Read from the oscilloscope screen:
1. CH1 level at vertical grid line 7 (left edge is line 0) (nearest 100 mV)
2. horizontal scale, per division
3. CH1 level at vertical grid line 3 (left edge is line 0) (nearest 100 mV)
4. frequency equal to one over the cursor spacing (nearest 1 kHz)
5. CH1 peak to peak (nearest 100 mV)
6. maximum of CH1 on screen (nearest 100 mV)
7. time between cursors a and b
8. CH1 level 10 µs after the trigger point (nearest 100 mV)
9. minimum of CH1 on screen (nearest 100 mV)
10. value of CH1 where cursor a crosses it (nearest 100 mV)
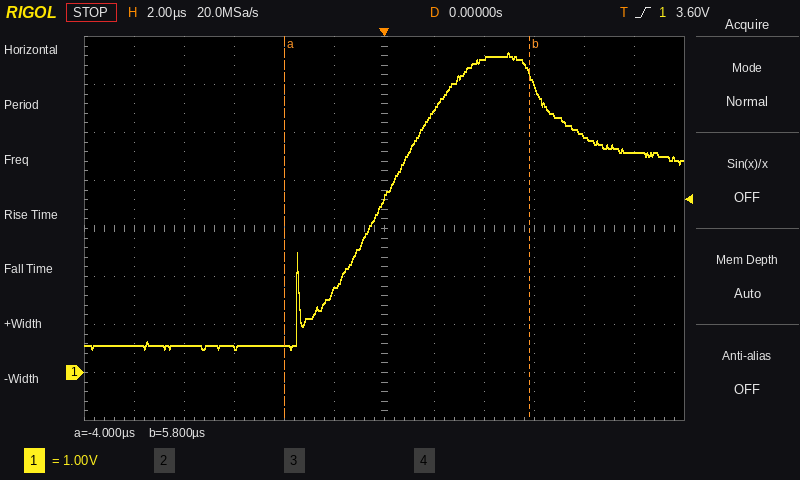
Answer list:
5.5 V
2 µs
500 mV
102 kHz
6.2 V
6.7 V
9.8 µs
4.6 V
500 mV
600 mV
